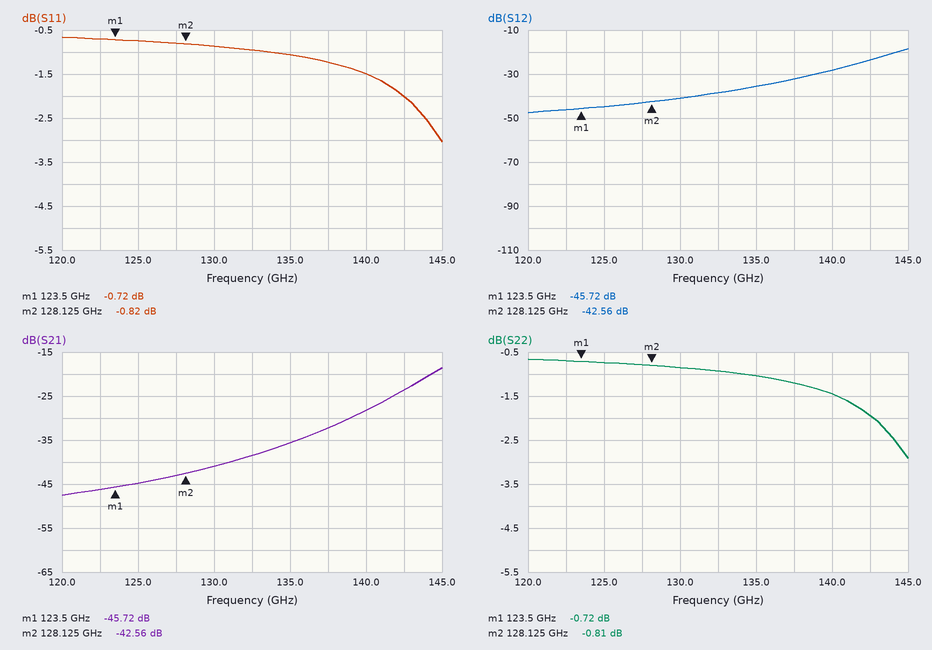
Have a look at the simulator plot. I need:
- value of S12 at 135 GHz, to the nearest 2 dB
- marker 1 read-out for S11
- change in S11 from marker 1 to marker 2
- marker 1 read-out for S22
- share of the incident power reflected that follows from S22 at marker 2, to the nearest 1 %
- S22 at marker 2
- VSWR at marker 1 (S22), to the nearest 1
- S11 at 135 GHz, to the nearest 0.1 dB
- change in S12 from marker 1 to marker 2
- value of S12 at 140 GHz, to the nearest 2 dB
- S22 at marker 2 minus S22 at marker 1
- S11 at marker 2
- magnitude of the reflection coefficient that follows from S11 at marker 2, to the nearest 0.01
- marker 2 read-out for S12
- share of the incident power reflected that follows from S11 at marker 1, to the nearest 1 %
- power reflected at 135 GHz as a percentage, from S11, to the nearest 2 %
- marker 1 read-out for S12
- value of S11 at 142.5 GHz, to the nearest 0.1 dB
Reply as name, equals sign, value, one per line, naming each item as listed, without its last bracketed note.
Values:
value of S12 at 135 GHz, to the nearest 2 dB = -36 dB
marker 1 read-out for S11 = -0.72 dB
change in S11 from marker 1 to marker 2 = -0.10 dB
marker 1 read-out for S22 = -0.72 dB
share of the incident power reflected that follows from S22 at marker 2, to the nearest 1 % = 83 %
S22 at marker 2 = -0.81 dB
VSWR at marker 1 (S22), to the nearest 1 = 24
S11 at 135 GHz, to the nearest 0.1 dB = -1.1 dB
change in S12 from marker 1 to marker 2 = 3.16 dB
value of S12 at 140 GHz, to the nearest 2 dB = -28 dB
S22 at marker 2 minus S22 at marker 1 = -0.09 dB
S11 at marker 2 = -0.82 dB
magnitude of the reflection coefficient that follows from S11 at marker 2, to the nearest 0.01 = 0.91
marker 2 read-out for S12 = -42.56 dB
share of the incident power reflected that follows from S11 at marker 1, to the nearest 1 % = 85 %
power reflected at 135 GHz as a percentage, from S11, to the nearest 2 % = 78 %
marker 1 read-out for S12 = -45.72 dB
value of S11 at 142.5 GHz, to the nearest 0.1 dB = -2.0 dB
